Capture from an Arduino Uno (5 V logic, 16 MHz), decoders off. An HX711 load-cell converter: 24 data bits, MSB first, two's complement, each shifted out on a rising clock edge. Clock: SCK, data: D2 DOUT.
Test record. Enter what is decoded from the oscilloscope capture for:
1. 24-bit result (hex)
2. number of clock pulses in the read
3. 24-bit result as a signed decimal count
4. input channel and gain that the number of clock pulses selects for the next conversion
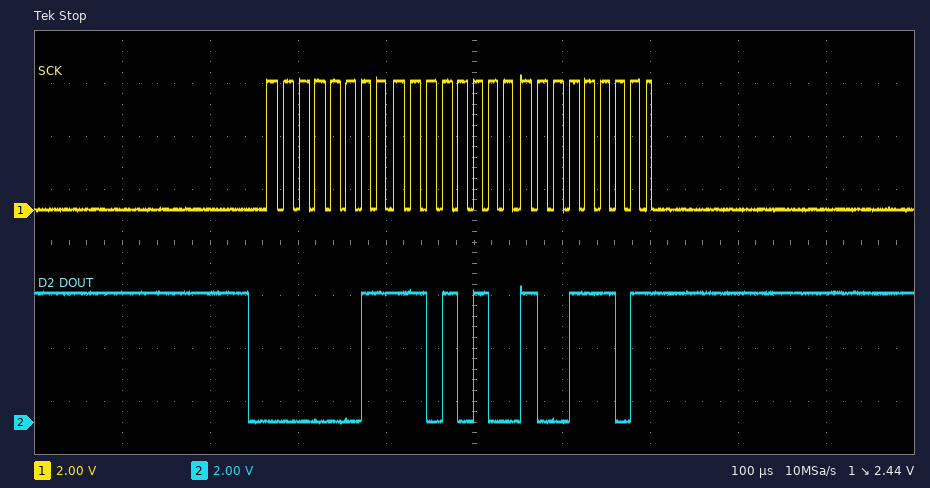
0x03D49D
25
251037
channel A, gain 128
